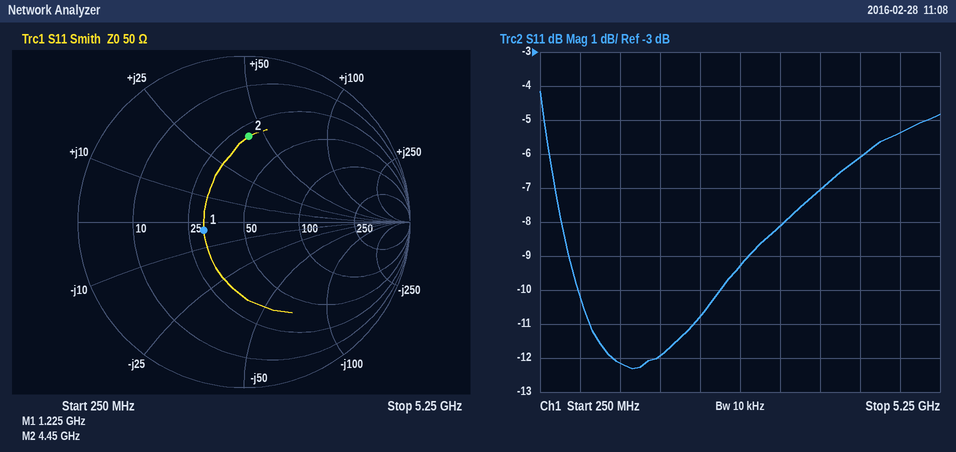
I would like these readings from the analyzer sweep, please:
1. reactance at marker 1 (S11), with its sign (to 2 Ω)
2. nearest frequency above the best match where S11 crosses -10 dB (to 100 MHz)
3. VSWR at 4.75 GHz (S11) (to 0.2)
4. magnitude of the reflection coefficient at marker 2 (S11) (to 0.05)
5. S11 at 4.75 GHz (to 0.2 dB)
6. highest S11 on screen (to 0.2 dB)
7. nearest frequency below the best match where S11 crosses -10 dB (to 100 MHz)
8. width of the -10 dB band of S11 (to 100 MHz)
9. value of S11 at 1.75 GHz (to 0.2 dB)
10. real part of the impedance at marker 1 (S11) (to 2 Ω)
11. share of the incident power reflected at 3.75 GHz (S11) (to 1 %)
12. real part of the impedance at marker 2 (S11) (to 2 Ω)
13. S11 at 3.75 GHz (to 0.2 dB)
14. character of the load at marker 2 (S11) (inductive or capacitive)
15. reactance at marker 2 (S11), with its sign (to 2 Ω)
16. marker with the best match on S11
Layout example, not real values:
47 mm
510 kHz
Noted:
-4 Ω
2.5 GHz
3.4
0.50
-5.4 dB
-4.2 dB
700 MHz
1.8 GHz
-12.0 dB
30 Ω
20 %
30 Ω
-7.0 dB
inductive
+42 Ω
marker 1
